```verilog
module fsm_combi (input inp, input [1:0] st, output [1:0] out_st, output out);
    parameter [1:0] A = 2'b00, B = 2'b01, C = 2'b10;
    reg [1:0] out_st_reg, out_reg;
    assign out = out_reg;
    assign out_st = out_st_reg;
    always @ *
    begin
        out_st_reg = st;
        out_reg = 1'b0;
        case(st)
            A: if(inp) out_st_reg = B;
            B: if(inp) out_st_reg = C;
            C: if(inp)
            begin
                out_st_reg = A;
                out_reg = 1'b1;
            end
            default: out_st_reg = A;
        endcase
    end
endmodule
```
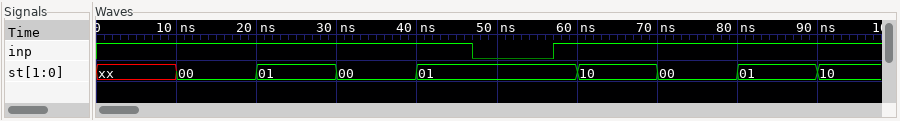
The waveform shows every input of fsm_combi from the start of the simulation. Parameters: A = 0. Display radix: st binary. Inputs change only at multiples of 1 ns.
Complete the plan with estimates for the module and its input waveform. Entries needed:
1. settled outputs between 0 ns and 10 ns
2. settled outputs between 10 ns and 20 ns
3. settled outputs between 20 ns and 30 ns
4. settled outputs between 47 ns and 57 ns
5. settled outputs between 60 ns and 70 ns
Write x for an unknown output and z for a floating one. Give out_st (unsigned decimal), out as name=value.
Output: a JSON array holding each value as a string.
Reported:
["out_st=0, out=0", "out_st=1, out=0", "out_st=2, out=0", "out_st=1, out=0", "out_st=0, out=1"]
